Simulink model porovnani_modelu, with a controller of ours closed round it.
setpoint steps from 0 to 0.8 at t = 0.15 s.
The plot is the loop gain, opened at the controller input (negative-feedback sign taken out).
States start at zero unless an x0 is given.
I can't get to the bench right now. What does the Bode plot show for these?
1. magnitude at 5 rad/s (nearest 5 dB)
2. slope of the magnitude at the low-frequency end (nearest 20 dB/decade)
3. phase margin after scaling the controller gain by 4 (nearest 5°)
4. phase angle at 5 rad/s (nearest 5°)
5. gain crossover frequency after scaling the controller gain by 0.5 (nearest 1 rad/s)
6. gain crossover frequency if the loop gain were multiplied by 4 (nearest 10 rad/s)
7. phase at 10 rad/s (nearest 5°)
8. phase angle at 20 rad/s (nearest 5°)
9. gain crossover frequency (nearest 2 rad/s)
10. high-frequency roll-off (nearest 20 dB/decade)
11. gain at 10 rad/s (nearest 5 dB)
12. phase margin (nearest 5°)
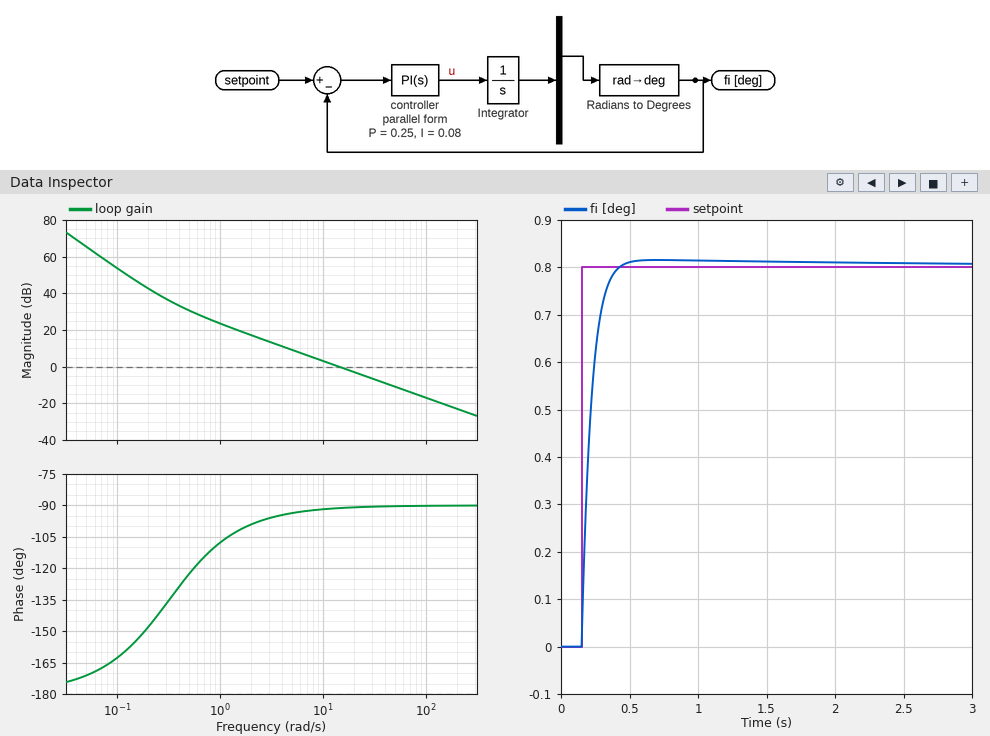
10 dB
-40 dB/decade
90°
-95°
7 rad/s
60 rad/s
-90°
-90°
14 rad/s
-20 dB/decade
5 dB
90°
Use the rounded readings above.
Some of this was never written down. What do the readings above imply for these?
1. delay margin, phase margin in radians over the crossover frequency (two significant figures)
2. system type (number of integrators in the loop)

0.11 s
2
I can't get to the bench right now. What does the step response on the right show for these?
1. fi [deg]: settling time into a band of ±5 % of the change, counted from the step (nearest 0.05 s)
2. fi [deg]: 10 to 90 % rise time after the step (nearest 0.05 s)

0.20 s
0.15 s
